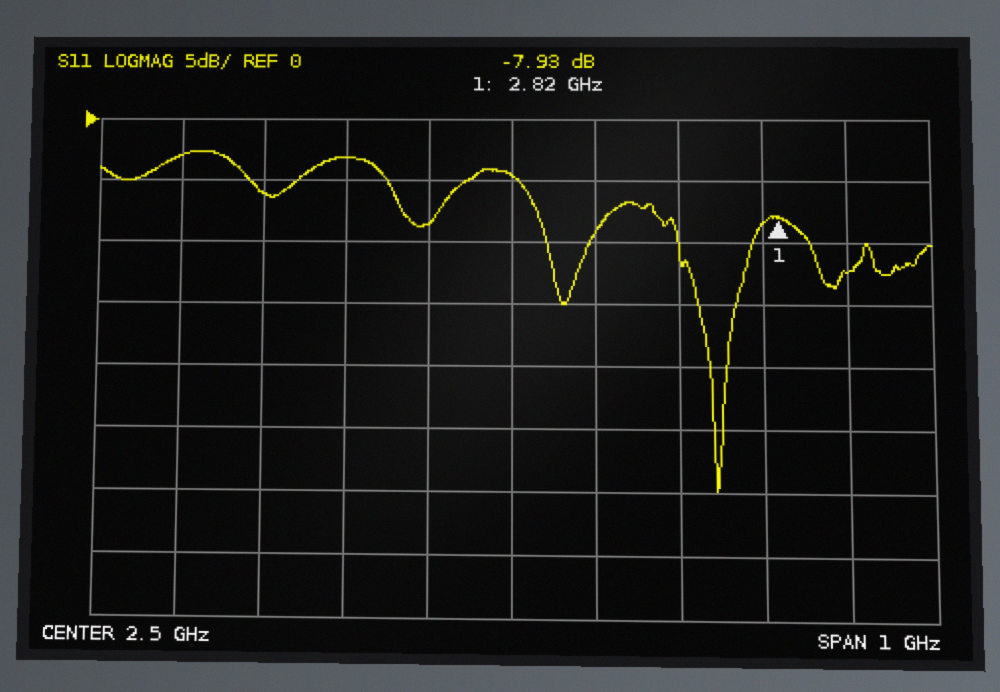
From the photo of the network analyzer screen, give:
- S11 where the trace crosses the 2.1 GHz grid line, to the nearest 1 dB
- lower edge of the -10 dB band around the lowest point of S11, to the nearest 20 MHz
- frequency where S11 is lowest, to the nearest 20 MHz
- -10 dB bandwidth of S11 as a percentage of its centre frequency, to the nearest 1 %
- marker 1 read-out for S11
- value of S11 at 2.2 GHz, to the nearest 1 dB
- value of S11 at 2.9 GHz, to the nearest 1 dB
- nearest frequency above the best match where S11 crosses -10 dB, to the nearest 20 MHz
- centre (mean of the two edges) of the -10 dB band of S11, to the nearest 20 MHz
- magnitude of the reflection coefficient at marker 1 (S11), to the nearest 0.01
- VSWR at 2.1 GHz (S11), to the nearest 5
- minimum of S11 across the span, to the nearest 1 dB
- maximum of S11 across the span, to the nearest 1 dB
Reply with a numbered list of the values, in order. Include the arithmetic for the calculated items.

1. -3 dB
2. 2.70 GHz
3. 2.74 GHz
4. 80 MHz / 2.74 GHz ≈ 3 %
5. -7.93 dB
6. -6 dB
7. -12 dB
8. 2.78 GHz
9. 2.74 GHz
10. 10^(-7.93/20) ≈ 0.40
11. |Γ| = 10^(-3/20) = 0.7079; VSWR = (1 + 0.7079)/(1 − 0.7079) ≈ 5.85, so 5 to the nearest 5
12. -30 dB
13. -3 dB
